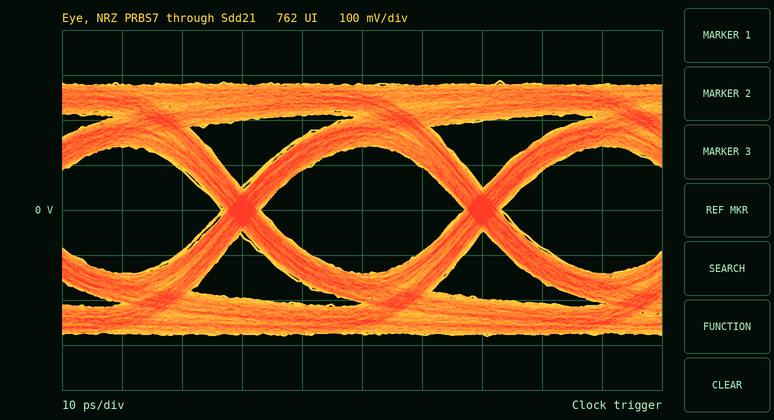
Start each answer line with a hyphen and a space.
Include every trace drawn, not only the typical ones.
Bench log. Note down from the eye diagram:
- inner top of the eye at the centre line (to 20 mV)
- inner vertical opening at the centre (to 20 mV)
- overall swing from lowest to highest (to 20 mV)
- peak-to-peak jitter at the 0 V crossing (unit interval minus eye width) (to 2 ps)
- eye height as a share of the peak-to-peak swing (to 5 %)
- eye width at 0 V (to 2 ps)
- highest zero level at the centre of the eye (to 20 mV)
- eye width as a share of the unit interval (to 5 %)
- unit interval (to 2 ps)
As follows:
- 140 mV
- 280 mV
- 560 mV
- 6 ps
- 50 %
- 34 ps
- -140 mV
- 85 %
- 40 ps
